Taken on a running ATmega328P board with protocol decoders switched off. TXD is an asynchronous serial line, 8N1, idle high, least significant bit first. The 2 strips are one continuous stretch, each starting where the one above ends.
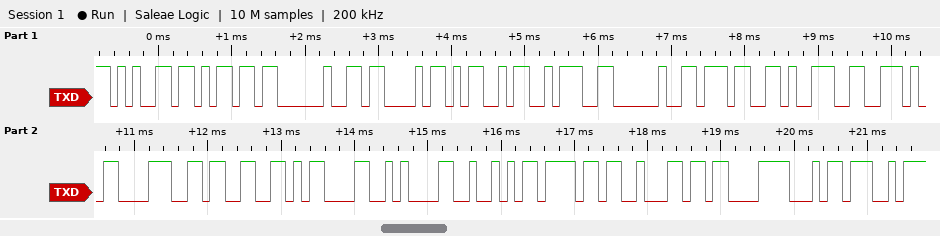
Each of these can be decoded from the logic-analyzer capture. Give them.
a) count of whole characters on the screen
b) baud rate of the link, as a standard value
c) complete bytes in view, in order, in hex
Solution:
19
9600 baud
0x65 0x6D 0x20 0x43 0x4D 0x3A 0x20 0x37 0x39 0x2E 0x38 0x33 0x0D 0x0A 0x52 0x6F 0x62 0xC3 0xB4
